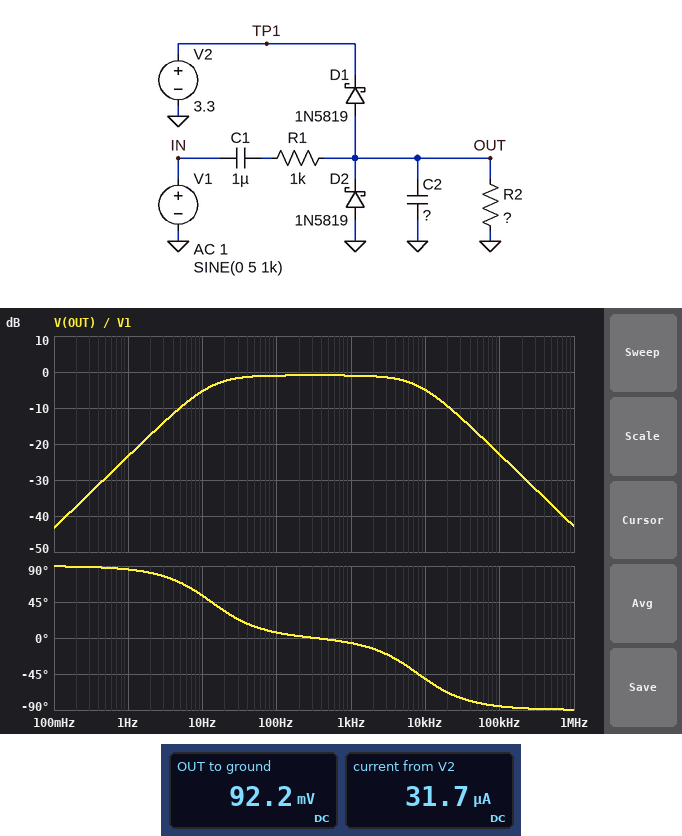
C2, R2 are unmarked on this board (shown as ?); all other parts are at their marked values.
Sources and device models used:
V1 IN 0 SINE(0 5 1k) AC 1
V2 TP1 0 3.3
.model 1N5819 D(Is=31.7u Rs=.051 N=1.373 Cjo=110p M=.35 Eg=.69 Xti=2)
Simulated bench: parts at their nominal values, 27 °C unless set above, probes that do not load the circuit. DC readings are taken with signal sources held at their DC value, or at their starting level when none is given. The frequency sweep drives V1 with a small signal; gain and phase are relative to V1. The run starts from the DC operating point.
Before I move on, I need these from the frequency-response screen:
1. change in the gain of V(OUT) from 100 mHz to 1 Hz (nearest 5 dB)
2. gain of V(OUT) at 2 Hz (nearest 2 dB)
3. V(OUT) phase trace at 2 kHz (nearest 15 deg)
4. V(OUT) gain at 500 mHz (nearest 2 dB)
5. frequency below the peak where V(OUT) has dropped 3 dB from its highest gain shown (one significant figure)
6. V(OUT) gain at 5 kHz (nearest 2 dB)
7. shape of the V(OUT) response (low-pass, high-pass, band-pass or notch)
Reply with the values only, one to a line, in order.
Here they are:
20 dB
-18 dB
-15 deg
-30 dB
10 Hz
-2 dB
band-pass
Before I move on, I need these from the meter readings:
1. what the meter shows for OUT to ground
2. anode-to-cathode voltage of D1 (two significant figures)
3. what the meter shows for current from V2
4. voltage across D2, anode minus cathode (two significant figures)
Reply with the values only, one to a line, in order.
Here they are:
92.2 mV
-3.2 V
31.7 µA
-92 mV
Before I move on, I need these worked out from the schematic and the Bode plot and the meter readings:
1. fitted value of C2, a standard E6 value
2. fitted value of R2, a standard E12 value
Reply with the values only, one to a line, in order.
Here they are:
22 nF
39 kΩ
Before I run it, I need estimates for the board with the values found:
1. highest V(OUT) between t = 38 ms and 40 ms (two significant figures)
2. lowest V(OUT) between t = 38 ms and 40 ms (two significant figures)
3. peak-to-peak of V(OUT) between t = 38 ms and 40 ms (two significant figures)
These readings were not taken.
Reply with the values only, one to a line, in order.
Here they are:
3.5 V
-160 mV
3.6 V
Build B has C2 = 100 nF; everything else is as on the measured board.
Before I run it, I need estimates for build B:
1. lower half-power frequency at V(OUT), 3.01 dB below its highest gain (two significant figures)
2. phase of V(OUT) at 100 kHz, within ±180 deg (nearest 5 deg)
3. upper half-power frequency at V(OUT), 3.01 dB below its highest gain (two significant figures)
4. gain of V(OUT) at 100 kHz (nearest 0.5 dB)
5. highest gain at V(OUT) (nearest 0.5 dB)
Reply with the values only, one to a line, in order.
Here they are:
12 Hz
-90 deg
1.9 kHz
-36.0 dB
-1.5 dB
